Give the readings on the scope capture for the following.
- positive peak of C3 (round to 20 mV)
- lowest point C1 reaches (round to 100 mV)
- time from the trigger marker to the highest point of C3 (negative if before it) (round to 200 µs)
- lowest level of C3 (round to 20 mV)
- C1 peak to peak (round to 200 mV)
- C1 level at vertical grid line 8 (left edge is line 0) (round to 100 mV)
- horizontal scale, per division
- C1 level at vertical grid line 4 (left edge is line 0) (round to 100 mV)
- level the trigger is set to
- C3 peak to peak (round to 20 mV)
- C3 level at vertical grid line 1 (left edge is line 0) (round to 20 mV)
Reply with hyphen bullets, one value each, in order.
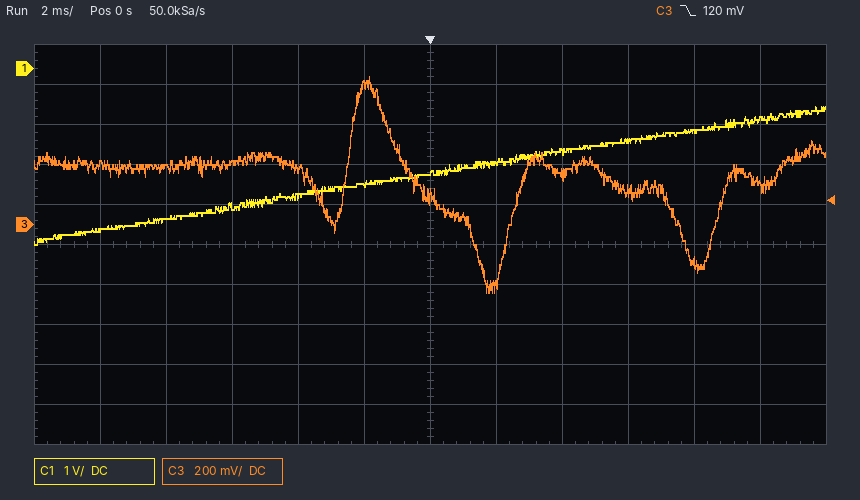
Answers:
- 740 mV
- -4.4 V
- -1.8 ms
- -340 mV
- 3.4 V
- -2.1 V
- 2 ms
- -3.2 V
- 120 mV
- 1.08 V
- 300 mV
